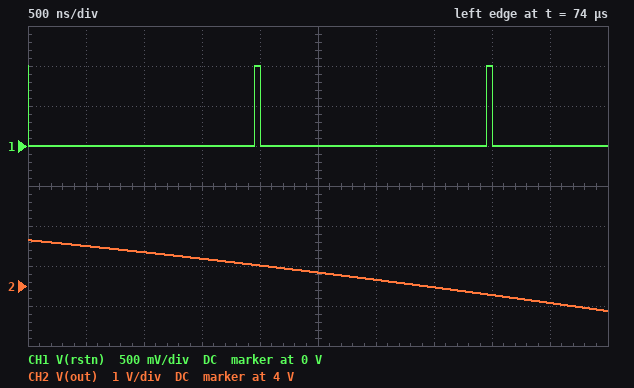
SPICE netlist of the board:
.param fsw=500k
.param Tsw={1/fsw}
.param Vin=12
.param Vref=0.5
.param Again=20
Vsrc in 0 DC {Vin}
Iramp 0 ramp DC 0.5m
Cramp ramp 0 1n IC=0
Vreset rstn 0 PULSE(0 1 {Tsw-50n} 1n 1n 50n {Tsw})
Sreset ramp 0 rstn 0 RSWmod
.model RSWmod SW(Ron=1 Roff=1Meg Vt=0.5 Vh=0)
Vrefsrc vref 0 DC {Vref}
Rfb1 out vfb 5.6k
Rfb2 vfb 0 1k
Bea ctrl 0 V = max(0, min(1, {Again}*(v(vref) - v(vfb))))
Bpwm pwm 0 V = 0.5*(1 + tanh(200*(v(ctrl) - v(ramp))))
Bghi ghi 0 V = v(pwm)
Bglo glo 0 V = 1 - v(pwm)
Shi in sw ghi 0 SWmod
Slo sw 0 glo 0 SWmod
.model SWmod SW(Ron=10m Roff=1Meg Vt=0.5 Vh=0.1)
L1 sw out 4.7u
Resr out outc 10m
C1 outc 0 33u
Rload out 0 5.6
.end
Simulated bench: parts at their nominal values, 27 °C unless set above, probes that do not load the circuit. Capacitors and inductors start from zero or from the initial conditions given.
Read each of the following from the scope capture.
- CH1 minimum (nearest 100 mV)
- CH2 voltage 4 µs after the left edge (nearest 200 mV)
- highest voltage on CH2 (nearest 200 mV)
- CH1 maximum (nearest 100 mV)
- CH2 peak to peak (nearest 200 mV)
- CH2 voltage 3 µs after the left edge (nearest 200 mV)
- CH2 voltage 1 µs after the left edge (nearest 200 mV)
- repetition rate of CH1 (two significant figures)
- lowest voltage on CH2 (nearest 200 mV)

0 V
3.8 V
5.2 V
1.0 V
1.8 V
4.2 V
4.8 V
500 kHz
3.4 V
